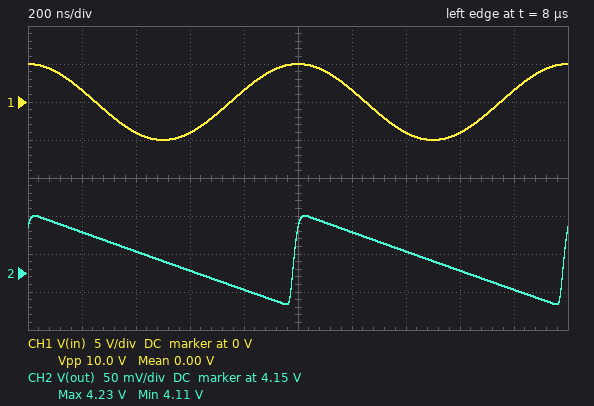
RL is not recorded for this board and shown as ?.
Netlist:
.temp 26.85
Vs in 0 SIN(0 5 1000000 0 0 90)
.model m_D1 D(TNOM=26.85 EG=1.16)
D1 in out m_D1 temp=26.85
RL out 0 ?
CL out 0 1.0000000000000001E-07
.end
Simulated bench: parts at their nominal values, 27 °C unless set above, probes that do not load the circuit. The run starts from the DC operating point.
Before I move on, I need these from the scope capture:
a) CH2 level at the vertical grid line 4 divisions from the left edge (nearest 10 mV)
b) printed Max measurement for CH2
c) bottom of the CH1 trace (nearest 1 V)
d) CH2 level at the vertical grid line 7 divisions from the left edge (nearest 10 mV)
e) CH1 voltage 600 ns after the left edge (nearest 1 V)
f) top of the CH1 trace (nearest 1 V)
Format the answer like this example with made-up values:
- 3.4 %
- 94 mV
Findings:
- 4.13 V
- 4.23 V
- -5 V
- 4.18 V
- -4 V
- 5 V
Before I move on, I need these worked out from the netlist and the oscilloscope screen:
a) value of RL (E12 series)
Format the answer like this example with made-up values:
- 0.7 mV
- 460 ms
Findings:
- 330 Ω
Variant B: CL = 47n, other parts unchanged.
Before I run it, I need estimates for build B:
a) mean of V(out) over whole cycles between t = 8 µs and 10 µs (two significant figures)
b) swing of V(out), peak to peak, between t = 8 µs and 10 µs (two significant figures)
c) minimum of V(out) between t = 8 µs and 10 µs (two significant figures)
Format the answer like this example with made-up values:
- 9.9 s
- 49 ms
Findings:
- 4.1 V
- 240 mV
- 4.0 V
